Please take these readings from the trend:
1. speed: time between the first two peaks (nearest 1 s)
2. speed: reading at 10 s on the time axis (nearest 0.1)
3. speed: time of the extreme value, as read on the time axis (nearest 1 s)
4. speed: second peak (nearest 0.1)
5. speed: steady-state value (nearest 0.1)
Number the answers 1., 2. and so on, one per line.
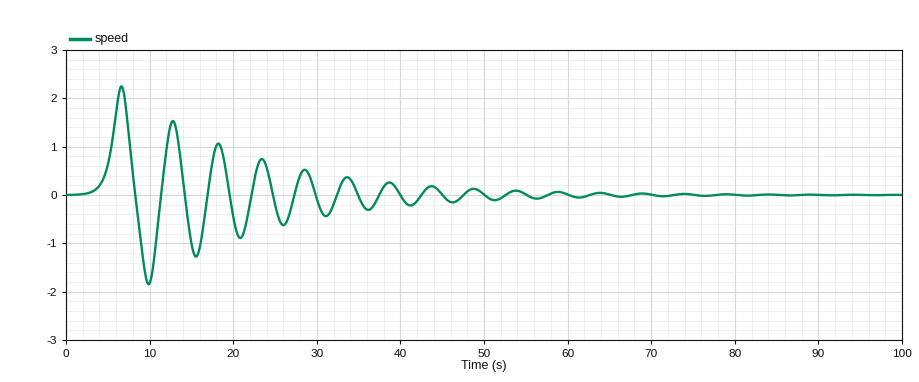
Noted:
1. 6 s
2. -1.8
3. 7 s
4. 1.5
5. 0.0
